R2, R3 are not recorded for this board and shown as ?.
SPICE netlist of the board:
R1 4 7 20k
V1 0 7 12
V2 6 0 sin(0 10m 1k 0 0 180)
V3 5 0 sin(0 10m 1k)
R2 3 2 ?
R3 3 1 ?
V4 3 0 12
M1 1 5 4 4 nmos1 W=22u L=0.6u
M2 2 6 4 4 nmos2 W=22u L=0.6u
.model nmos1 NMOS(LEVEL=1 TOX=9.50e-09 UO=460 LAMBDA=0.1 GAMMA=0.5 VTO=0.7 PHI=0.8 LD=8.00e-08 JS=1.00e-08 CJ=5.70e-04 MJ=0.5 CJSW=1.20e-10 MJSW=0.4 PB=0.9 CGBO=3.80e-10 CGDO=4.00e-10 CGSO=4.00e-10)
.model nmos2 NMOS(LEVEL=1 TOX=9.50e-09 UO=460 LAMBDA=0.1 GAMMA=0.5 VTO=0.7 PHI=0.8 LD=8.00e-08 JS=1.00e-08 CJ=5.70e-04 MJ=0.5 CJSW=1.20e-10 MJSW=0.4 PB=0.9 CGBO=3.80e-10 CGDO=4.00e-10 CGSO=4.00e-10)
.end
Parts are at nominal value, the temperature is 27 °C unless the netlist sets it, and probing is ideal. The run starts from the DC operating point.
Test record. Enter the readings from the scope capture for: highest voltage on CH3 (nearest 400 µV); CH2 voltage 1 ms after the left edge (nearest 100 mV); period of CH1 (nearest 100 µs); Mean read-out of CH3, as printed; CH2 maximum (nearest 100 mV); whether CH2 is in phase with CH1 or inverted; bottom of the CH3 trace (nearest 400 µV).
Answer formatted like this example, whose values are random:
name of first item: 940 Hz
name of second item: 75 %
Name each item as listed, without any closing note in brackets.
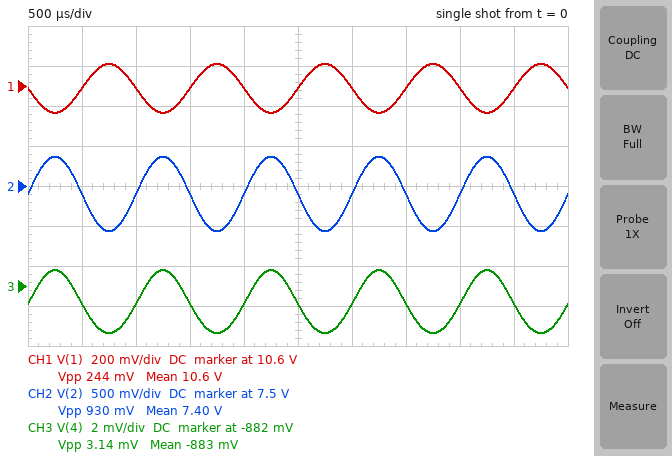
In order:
highest voltage on CH3: -881.2 mV
CH2 voltage 1 ms after the left edge: 7.4 V
period of CH1: 1.0 ms
Mean read-out of CH3, as printed: -883 mV
CH2 maximum: 7.9 V
whether CH2 is in phase with CH1 or inverted: inverted
bottom of the CH3 trace: -884.4 mV
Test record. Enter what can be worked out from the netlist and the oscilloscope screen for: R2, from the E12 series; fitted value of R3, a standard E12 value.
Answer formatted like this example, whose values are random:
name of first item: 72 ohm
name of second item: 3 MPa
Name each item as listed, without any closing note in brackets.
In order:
R2, from the E12 series: 18 kΩ
fitted value of R3, a standard E12 value: 4.7 kΩ
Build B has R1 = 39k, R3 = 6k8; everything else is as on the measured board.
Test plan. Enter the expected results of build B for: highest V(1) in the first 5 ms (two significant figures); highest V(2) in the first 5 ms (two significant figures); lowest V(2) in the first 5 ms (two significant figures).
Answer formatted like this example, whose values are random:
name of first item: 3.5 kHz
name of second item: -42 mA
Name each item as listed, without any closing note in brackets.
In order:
highest V(1) in the first 5 ms: 11 V
highest V(2) in the first 5 ms: 9.9 V
lowest V(2) in the first 5 ms: 9.1 V
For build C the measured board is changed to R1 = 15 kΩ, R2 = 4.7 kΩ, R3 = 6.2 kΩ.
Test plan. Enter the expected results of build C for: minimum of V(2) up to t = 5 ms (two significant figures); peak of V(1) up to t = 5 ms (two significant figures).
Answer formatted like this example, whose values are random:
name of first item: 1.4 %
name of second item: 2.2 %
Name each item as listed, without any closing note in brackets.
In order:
minimum of V(2) up to t = 5 ms: 10 V
peak of V(1) up to t = 5 ms: 9.9 V
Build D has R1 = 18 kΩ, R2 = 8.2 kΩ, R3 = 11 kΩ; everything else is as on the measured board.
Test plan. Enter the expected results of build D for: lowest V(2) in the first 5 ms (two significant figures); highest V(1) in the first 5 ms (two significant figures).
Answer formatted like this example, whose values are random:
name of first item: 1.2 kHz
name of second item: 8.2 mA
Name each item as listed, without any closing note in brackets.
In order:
lowest V(2) in the first 5 ms: 9.2 V
highest V(1) in the first 5 ms: 9.0 V
